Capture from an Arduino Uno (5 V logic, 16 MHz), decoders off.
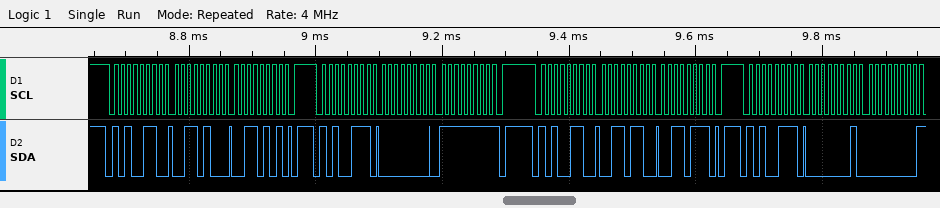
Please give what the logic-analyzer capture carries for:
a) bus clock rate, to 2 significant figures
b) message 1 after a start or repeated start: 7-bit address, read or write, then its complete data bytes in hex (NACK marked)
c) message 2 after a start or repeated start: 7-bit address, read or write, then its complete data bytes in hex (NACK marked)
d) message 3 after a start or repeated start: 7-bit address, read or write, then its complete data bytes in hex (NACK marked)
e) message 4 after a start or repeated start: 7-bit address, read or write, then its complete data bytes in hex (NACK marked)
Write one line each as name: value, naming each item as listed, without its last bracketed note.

bus clock rate, to 2 significant figures: 100 kHz
message 1 after a start or repeated start: 7-bit address, read or write, then its complete data bytes in hex: 0x53 write: 34 35
message 2 after a start or repeated start: 7-bit address, read or write, then its complete data bytes in hex: 0x53 read: 00 FF NACK
message 3 after a start or repeated start: 7-bit address, read or write, then its complete data bytes in hex: 0x53 write: 36 37
message 4 after a start or repeated start: 7-bit address, read or write, then its complete data bytes in hex: 0x53 read: 01 00 NACK
